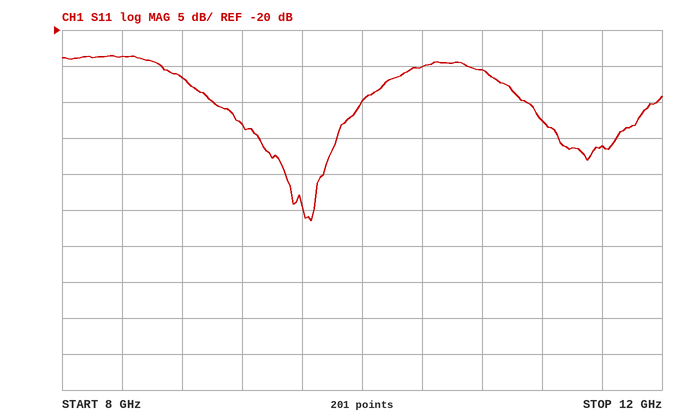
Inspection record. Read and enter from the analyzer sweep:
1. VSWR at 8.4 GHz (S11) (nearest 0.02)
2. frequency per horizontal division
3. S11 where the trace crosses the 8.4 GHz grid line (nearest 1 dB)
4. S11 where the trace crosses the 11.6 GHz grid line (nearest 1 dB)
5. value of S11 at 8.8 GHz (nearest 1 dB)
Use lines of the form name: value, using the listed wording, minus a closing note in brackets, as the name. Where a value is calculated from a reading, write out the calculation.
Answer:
VSWR at 8.4 GHz (S11): |Γ| = 10^(-24/20) = 0.0631; VSWR = (1 + 0.0631)/(1 − 0.0631) ≈ 1.13, so 1.14 to the nearest 0.02
frequency per horizontal division: 400 MHz
S11 where the trace crosses the 8.4 GHz grid line: -24 dB
S11 where the trace crosses the 11.6 GHz grid line: -36 dB
value of S11 at 8.8 GHz: -27 dB
